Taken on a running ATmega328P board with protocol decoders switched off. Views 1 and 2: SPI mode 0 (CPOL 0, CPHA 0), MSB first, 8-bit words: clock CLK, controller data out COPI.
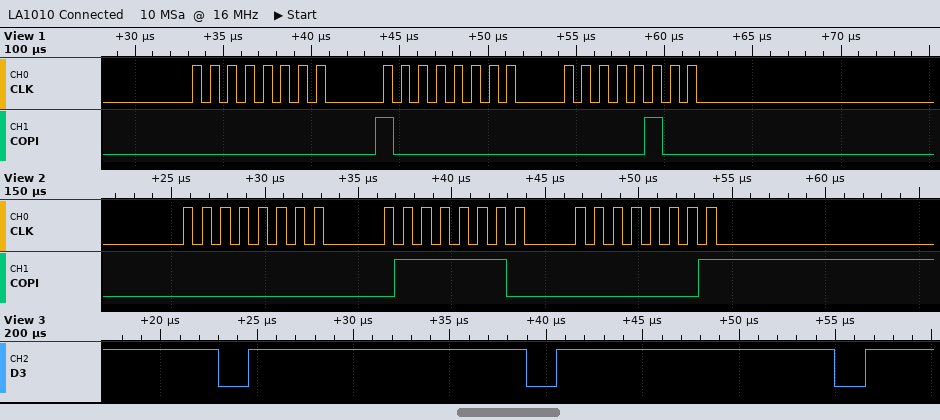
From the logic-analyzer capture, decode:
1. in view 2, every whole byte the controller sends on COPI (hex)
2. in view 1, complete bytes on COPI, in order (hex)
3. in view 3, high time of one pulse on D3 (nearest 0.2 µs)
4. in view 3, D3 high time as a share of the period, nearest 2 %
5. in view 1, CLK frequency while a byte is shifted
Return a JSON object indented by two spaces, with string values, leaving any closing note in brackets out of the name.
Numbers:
{
  "in view 2, every whole byte the controller sends on COPI": "0x00 0x7E 0x01",
  "in view 1, complete bytes on COPI, in order": "00 80 04",
  "in view 3, high time of one pulse on D3": "14.4 µs",
  "in view 3, D3 high time as a share of the period, nearest 2 %": "90 %",
  "in view 1, CLK frequency while a byte is shifted": "1 MHz"
}
